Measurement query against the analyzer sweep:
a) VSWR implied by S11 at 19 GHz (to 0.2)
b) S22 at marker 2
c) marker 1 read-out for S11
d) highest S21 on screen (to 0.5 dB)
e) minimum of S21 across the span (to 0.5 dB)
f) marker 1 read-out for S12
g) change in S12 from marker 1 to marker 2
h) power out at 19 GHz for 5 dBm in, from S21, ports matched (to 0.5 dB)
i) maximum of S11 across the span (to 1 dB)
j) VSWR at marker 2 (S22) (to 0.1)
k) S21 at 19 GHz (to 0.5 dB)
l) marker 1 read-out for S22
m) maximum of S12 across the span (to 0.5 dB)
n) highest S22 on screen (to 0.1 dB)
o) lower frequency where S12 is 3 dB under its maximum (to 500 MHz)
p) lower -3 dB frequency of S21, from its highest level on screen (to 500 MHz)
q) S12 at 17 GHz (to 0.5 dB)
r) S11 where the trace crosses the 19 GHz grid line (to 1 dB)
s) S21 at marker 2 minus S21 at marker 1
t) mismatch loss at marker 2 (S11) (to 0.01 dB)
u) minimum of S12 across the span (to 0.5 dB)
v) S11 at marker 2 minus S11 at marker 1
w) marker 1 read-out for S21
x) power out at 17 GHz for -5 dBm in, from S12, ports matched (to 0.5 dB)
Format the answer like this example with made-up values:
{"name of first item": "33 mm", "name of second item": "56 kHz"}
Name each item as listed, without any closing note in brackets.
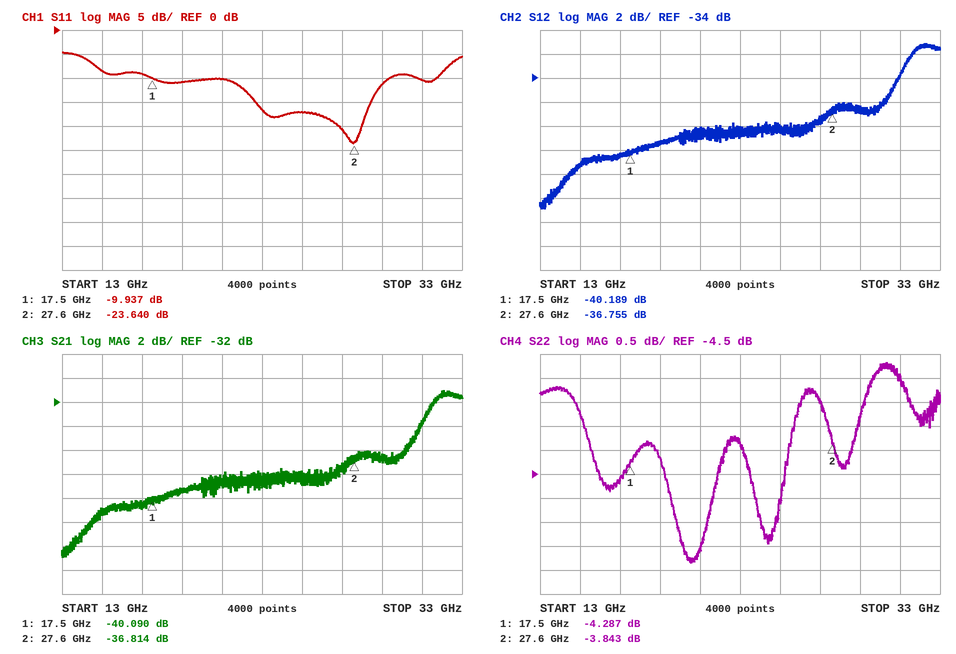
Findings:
{"VSWR implied by S11 at 19 GHz": "1.8", "S22 at marker 2": "-3.843 dB", "marker 1 read-out for S11": "-9.937 dB", "highest S21 on screen": "-31.0 dB", "minimum of S21 across the span": "-45.0 dB", "marker 1 read-out for S12": "-40.189 dB", "change in S12 from marker 1 to marker 2": "3.434 dB", "power out at 19 GHz for 5 dBm in, from S21, ports matched": "-34.5 dBm", "maximum of S11 across the span": "-5 dB", "VSWR at marker 2 (S22)": "4.6", "S21 at 19 GHz": "-39.5 dB", "marker 1 read-out for S22": "-4.287 dB", "maximum of S12 across the span": "-31.0 dB", "highest S22 on screen": "-2.2 dB", "lower frequency where S12 is 3 dB under its maximum": "31.0 GHz", "lower -3 dB frequency of S21, from its highest level on screen": "31.0 GHz", "S12 at 17 GHz": "-40.5 dB", "S11 where the trace crosses the 19 GHz grid line": "-11 dB", "S21 at marker 2 minus S21 at marker 1": "3.276 dB", "mismatch loss at marker 2 (S11)": "0.02 dB", "minimum of S12 across the span": "-45.0 dB", "S11 at marker 2 minus S11 at marker 1": "-13.703 dB", "marker 1 read-out for S21": "-40.090 dB", "power out at 17 GHz for -5 dBm in, from S12, ports matched": "-45.5 dBm"}
